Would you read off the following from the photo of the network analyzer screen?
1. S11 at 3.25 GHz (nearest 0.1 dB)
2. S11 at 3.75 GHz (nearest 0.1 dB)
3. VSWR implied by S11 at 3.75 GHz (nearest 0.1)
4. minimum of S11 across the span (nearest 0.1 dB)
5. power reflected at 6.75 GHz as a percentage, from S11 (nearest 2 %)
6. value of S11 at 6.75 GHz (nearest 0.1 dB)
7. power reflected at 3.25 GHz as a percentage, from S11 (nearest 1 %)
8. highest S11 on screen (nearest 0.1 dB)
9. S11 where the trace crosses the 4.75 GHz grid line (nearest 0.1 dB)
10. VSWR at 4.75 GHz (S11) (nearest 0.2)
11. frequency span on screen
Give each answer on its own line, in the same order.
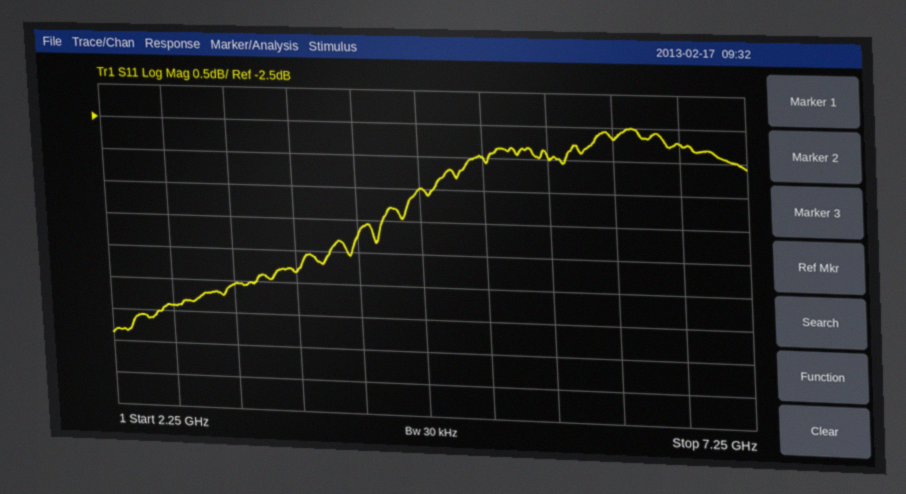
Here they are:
-5.1 dB
-4.8 dB
3.7
-5.9 dB
54 %
-2.7 dB
31 %
-2.5 dB
-3.5 dB
5.0
5 GHz
